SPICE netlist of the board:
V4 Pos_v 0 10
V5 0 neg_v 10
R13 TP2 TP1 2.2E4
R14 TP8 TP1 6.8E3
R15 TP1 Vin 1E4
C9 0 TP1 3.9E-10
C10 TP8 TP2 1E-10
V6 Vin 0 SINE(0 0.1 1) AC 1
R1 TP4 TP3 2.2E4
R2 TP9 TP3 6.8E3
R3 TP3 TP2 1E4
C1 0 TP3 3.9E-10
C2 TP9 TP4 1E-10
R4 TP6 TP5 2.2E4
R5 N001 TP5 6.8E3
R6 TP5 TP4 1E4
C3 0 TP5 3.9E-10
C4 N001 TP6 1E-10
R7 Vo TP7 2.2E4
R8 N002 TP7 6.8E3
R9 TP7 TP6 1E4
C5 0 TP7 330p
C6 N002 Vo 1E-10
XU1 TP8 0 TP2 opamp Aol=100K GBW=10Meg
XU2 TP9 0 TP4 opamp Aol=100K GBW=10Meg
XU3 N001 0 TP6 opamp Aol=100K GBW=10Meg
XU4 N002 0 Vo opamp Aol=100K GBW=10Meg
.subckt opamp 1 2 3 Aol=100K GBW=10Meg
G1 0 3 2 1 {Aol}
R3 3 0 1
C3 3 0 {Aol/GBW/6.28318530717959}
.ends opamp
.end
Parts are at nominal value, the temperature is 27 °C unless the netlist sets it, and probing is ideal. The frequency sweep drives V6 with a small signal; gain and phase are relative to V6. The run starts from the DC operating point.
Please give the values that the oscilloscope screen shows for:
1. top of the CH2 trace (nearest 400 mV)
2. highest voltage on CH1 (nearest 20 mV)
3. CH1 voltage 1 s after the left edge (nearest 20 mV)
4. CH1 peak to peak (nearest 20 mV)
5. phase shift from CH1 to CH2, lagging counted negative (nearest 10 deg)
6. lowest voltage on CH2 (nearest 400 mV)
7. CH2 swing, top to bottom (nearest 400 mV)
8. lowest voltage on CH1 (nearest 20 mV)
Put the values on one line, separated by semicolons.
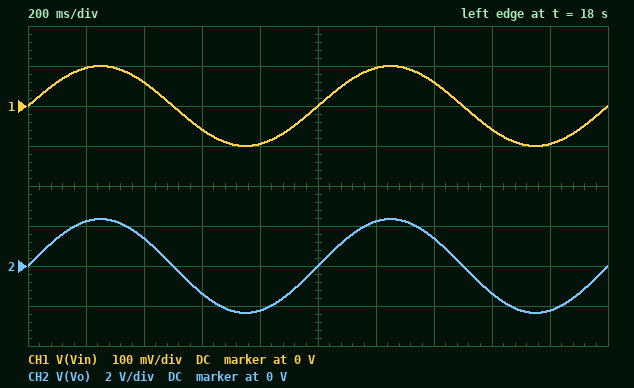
2.4 V; 100 mV; 0 V; 200 mV; 0 deg; -2.4 V; 4.8 V; -100 mV
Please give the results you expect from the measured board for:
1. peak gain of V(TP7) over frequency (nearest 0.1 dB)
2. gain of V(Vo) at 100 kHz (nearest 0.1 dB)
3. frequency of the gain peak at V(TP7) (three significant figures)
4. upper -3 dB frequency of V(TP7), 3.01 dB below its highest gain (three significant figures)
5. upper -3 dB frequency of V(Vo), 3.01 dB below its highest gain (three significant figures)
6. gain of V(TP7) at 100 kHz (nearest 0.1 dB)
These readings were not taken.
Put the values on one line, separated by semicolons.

4.9 dB; -11.4 dB; 28.4 kHz; 47.7 kHz; 23.5 kHz; -18.5 dB
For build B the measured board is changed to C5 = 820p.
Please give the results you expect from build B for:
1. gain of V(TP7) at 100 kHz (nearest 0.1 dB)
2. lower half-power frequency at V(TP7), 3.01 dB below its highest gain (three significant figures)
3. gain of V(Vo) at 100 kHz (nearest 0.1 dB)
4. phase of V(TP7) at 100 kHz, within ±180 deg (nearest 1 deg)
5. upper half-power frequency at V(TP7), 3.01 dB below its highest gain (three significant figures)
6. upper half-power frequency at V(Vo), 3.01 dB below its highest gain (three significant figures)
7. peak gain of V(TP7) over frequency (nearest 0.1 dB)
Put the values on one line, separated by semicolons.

-22.8 dB; 15.4 kHz; -15.7 dB; 135 deg; 45.8 kHz; 28.1 kHz; 6.2 dB
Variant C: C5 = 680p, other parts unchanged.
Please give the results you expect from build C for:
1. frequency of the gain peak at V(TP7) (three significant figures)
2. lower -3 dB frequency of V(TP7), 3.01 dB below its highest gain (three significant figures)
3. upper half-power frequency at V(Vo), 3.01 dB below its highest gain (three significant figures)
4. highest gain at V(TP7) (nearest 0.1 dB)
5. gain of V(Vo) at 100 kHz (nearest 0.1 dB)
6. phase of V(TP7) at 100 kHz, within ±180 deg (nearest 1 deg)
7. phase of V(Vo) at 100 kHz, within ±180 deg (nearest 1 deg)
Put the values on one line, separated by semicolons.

29.7 kHz; 14.9 kHz; 26.7 kHz; 5.8 dB; -14.4 dB; 142 deg; -129 deg
